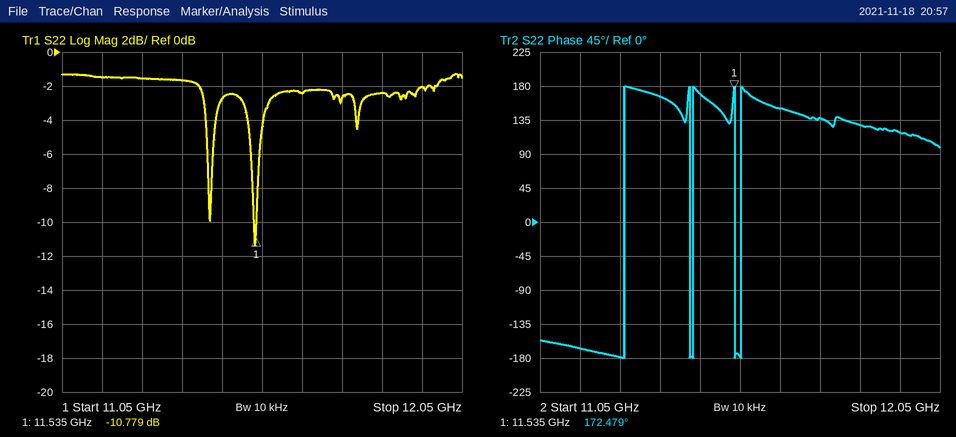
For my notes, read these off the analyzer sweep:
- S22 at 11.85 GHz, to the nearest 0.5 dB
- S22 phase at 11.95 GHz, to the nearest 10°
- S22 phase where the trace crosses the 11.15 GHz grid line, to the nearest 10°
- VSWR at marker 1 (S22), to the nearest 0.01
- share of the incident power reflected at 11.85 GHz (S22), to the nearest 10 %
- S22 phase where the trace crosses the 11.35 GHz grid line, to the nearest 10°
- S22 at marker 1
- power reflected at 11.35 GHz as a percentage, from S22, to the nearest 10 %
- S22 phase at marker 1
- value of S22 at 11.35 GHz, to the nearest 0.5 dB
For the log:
-2.5 dB
120°
-170°
1.81
60 %
170°
-10.779 dB
70 %
172.479°
-1.5 dB
